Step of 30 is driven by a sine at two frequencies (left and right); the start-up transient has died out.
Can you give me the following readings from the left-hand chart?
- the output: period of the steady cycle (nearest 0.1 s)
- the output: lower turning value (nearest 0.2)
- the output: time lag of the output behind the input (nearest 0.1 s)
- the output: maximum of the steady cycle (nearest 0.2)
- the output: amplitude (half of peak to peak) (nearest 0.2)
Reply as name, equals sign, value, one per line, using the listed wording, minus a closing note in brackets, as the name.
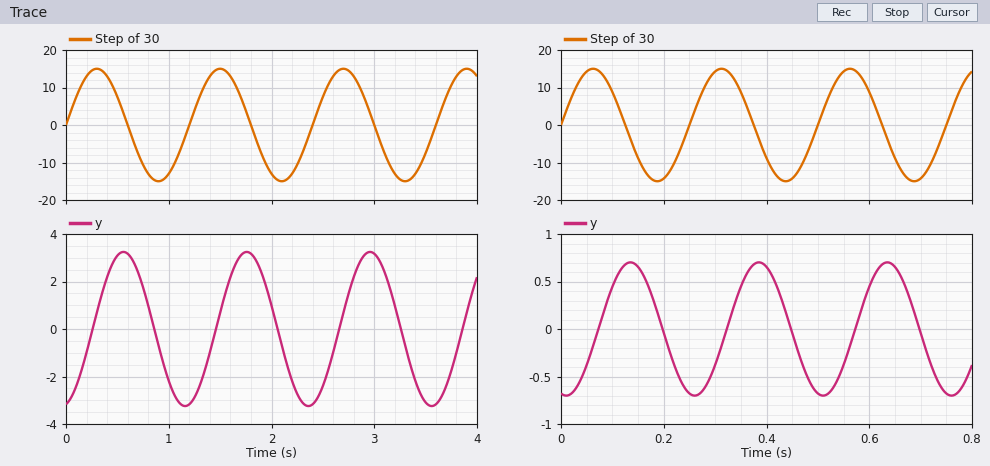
the output: period of the steady cycle = 1.2 s
the output: lower turning value = -3.2
the output: time lag of the output behind the input = 0.3 s
the output: maximum of the steady cycle = 3.2
the output: amplitude (half of peak to peak) = 3.2
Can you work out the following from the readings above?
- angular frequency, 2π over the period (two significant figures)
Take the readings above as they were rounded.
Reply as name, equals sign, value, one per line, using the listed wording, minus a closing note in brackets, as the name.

angular frequency, 2π over the period = 5.2 rad/s
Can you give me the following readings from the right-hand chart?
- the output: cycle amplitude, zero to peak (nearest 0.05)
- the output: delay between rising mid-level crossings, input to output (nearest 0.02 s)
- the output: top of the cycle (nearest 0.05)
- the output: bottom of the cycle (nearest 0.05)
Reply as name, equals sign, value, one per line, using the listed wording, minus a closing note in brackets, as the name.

the output: cycle amplitude, zero to peak = 0.70
the output: delay between rising mid-level crossings, input to output = 0.08 s
the output: top of the cycle = 0.70
the output: bottom of the cycle = -0.70
